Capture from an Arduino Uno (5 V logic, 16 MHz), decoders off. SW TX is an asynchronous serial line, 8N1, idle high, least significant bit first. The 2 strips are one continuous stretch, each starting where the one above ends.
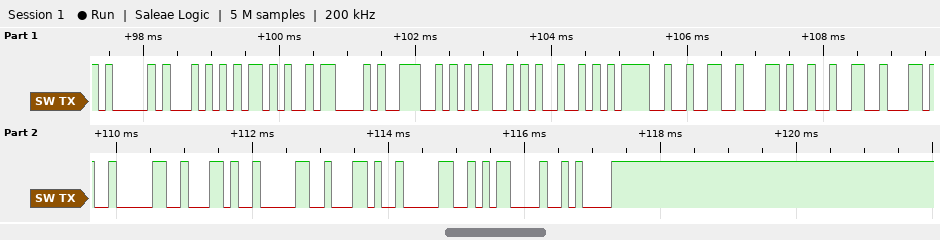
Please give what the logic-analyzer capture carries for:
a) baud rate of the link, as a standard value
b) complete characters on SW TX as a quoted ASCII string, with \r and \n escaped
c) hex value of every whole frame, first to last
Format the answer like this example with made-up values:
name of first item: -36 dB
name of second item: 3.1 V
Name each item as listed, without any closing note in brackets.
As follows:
baud rate of the link, as a standard value: 9600 baud
complete characters on SW TX as a quoted ASCII string, with \r and \n escaped: "AT+CNMI=2,2,0,0,0\r\n"
hex value of every whole frame, first to last: 0x41 0x54 0x2B 0x43 0x4E 0x4D 0x49 0x3D 0x32 0x2C 0x32 0x2C 0x30 0x2C 0x30 0x2C 0x30 0x0D 0x0A
